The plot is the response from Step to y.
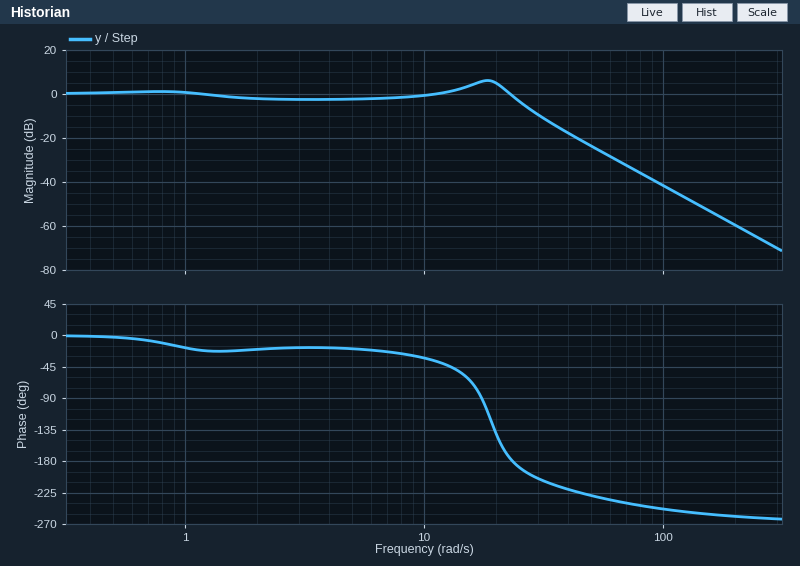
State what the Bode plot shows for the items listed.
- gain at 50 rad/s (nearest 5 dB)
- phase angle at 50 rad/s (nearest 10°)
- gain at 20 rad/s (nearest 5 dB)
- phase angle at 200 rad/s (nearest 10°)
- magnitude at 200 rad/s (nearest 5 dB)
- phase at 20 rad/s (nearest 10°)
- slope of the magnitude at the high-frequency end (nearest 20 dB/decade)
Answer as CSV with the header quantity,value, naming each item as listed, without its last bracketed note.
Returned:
quantity,value
gain at 50 rad/s,-25 dB
phase angle at 50 rad/s,-230°
gain at 20 rad/s,5 dB
phase angle at 200 rad/s,-260°
magnitude at 200 rad/s,-60 dB
phase at 20 rad/s,-140°
slope of the magnitude at the high-frequency end,-60 dB/decade
